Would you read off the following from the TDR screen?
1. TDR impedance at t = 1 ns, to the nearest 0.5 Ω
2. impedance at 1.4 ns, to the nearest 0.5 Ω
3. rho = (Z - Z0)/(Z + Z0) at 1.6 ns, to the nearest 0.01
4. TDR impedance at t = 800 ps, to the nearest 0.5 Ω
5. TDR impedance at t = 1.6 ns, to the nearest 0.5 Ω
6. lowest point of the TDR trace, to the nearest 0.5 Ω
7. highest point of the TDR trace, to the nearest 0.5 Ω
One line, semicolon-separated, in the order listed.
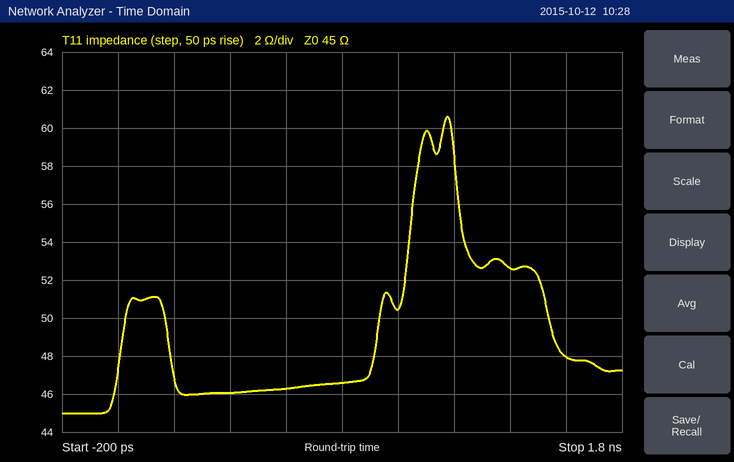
50.5 Ω; 52.5 Ω; +0.03; 46.5 Ω; 48.0 Ω; 45.0 Ω; 60.5 Ω
